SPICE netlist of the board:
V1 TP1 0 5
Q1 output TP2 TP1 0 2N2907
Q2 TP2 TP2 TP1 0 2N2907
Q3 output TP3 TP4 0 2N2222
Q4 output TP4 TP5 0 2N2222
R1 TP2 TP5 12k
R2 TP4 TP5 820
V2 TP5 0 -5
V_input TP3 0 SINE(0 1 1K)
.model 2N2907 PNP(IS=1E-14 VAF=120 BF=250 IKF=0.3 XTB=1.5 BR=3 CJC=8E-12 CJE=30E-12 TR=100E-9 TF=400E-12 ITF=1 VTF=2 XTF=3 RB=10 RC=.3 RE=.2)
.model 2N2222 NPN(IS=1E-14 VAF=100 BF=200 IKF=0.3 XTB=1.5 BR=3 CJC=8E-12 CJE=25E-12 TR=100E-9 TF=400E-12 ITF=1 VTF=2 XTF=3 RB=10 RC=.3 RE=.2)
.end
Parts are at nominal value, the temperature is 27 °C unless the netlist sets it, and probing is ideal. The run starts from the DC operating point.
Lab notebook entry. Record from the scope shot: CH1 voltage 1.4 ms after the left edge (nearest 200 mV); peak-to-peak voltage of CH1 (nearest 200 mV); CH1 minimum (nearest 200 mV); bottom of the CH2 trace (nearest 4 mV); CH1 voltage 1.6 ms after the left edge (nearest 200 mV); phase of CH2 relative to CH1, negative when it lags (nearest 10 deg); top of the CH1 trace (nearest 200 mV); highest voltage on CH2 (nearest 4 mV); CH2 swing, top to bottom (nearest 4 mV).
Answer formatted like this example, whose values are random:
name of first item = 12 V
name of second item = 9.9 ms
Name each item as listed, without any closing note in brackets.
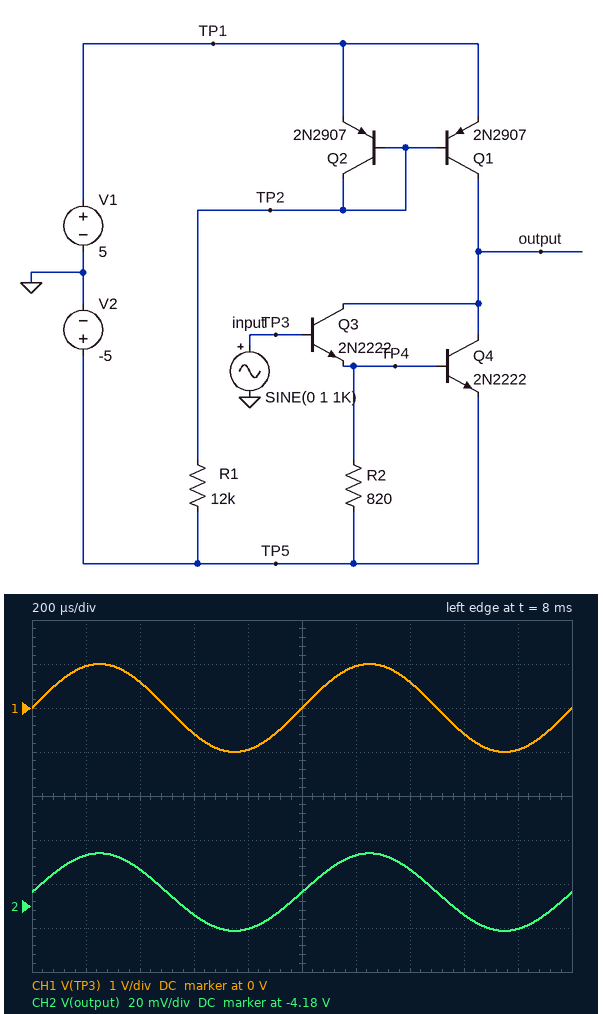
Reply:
CH1 voltage 1.4 ms after the left edge = 600 mV
peak-to-peak voltage of CH1 = 2.0 V
CH1 minimum = -1.0 V
bottom of the CH2 trace = -4.192 V
CH1 voltage 1.6 ms after the left edge = -600 mV
phase of CH2 relative to CH1, negative when it lags = 0 deg
top of the CH1 trace = 1.0 V
highest voltage on CH2 = -4.156 V
CH2 swing, top to bottom = 36 mV
